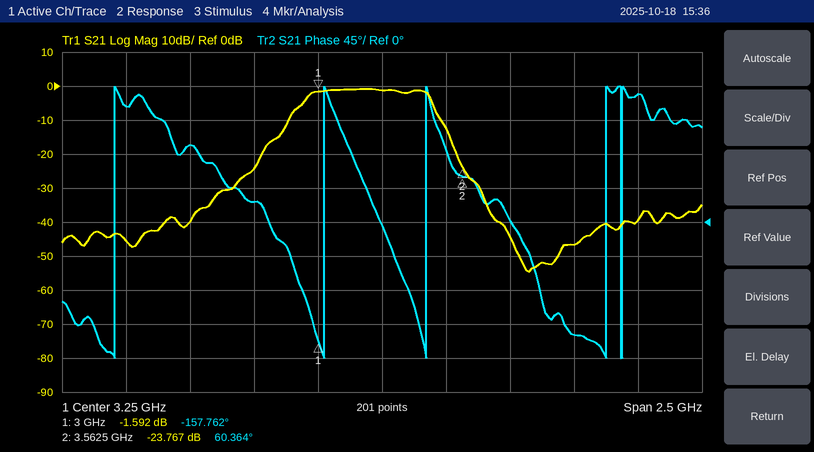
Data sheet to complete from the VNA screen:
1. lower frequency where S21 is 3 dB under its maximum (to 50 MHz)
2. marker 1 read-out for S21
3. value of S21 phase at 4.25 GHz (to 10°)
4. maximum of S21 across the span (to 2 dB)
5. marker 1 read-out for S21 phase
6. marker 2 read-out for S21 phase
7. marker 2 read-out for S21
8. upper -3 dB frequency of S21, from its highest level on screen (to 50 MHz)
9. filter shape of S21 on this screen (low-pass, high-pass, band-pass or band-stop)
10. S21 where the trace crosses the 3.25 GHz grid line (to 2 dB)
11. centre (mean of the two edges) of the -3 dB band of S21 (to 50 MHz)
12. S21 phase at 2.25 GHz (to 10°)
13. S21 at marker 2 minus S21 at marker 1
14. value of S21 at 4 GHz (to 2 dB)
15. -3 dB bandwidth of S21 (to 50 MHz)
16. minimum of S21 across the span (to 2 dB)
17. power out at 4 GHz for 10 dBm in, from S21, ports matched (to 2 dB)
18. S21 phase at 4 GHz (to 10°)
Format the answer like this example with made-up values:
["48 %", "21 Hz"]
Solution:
["2.95 GHz", "-1.592 dB", "170°", "0 dB", "-157.762°", "60.364°", "-23.767 dB", "3.45 GHz", "band-pass", "-2 dB", "3.20 GHz", "150°", "-22.175 dB", "-46 dB", "500 MHz", "-54 dB", "-36 dBm", "-150°"]
